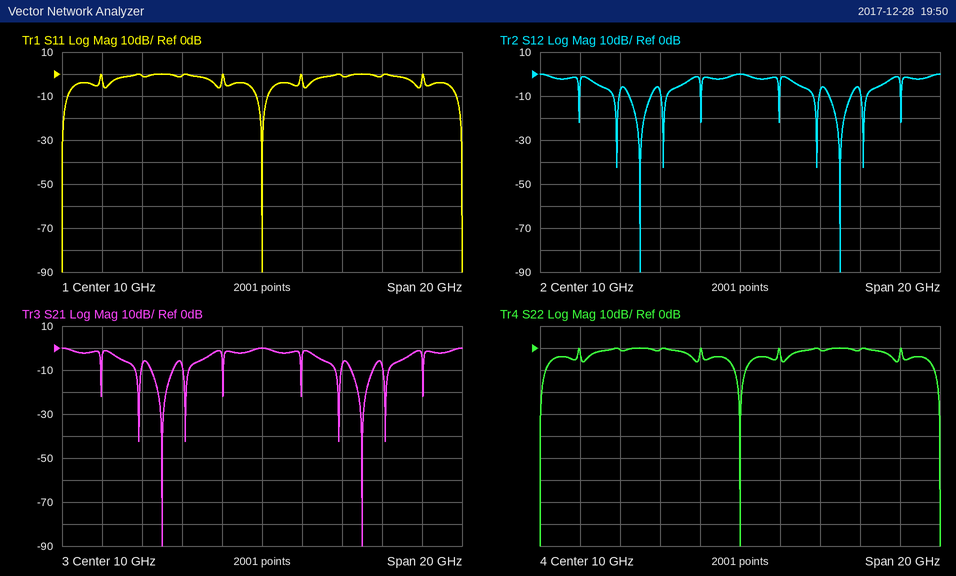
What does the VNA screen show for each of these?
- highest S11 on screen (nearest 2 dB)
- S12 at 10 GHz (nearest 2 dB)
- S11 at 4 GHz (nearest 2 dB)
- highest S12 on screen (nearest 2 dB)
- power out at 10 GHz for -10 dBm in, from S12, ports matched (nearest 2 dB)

0 dB
0 dB
0 dB
0 dB
-10 dBm
